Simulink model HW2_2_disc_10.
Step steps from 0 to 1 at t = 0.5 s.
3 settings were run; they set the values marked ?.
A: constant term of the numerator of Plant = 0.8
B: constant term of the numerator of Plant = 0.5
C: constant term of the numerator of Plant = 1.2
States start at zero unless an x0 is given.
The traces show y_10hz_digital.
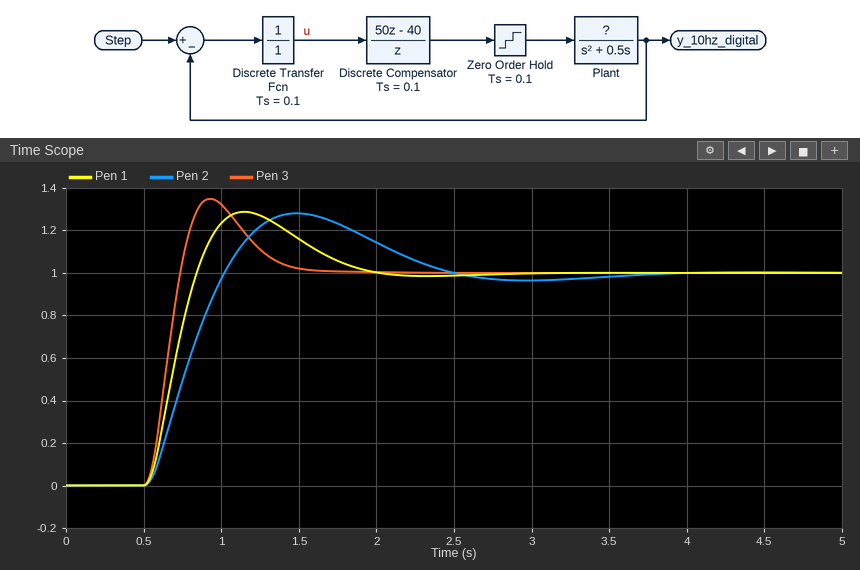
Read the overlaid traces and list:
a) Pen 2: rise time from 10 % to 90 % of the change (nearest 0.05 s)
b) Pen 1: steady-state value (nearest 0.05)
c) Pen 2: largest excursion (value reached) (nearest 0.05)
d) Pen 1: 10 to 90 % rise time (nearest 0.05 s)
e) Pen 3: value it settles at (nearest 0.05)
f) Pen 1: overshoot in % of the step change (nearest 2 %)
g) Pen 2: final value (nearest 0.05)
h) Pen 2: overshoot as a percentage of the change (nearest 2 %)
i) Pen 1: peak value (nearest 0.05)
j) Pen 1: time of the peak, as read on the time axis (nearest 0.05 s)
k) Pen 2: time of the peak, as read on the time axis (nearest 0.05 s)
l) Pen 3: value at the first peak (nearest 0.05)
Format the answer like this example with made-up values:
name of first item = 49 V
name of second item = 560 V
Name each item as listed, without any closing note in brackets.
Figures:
Pen 2: rise time from 10 % to 90 % of the change = 0.35 s
Pen 1: steady-state value = 1.00
Pen 2: largest excursion (value reached) = 1.30
Pen 1: 10 to 90 % rise time = 0.25 s
Pen 3: value it settles at = 1.00
Pen 1: overshoot in % of the step change = 28 %
Pen 2: final value = 1.00
Pen 2: overshoot as a percentage of the change = 28 %
Pen 1: peak value = 1.30
Pen 1: time of the peak, as read on the time axis = 1.15 s
Pen 2: time of the peak, as read on the time axis = 1.50 s
Pen 3: value at the first peak = 1.35
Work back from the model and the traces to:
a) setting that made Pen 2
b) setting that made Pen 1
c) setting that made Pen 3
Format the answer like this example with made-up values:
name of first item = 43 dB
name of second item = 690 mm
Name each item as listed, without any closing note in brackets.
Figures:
setting that made Pen 2 = B
setting that made Pen 1 = A
setting that made Pen 3 = C
